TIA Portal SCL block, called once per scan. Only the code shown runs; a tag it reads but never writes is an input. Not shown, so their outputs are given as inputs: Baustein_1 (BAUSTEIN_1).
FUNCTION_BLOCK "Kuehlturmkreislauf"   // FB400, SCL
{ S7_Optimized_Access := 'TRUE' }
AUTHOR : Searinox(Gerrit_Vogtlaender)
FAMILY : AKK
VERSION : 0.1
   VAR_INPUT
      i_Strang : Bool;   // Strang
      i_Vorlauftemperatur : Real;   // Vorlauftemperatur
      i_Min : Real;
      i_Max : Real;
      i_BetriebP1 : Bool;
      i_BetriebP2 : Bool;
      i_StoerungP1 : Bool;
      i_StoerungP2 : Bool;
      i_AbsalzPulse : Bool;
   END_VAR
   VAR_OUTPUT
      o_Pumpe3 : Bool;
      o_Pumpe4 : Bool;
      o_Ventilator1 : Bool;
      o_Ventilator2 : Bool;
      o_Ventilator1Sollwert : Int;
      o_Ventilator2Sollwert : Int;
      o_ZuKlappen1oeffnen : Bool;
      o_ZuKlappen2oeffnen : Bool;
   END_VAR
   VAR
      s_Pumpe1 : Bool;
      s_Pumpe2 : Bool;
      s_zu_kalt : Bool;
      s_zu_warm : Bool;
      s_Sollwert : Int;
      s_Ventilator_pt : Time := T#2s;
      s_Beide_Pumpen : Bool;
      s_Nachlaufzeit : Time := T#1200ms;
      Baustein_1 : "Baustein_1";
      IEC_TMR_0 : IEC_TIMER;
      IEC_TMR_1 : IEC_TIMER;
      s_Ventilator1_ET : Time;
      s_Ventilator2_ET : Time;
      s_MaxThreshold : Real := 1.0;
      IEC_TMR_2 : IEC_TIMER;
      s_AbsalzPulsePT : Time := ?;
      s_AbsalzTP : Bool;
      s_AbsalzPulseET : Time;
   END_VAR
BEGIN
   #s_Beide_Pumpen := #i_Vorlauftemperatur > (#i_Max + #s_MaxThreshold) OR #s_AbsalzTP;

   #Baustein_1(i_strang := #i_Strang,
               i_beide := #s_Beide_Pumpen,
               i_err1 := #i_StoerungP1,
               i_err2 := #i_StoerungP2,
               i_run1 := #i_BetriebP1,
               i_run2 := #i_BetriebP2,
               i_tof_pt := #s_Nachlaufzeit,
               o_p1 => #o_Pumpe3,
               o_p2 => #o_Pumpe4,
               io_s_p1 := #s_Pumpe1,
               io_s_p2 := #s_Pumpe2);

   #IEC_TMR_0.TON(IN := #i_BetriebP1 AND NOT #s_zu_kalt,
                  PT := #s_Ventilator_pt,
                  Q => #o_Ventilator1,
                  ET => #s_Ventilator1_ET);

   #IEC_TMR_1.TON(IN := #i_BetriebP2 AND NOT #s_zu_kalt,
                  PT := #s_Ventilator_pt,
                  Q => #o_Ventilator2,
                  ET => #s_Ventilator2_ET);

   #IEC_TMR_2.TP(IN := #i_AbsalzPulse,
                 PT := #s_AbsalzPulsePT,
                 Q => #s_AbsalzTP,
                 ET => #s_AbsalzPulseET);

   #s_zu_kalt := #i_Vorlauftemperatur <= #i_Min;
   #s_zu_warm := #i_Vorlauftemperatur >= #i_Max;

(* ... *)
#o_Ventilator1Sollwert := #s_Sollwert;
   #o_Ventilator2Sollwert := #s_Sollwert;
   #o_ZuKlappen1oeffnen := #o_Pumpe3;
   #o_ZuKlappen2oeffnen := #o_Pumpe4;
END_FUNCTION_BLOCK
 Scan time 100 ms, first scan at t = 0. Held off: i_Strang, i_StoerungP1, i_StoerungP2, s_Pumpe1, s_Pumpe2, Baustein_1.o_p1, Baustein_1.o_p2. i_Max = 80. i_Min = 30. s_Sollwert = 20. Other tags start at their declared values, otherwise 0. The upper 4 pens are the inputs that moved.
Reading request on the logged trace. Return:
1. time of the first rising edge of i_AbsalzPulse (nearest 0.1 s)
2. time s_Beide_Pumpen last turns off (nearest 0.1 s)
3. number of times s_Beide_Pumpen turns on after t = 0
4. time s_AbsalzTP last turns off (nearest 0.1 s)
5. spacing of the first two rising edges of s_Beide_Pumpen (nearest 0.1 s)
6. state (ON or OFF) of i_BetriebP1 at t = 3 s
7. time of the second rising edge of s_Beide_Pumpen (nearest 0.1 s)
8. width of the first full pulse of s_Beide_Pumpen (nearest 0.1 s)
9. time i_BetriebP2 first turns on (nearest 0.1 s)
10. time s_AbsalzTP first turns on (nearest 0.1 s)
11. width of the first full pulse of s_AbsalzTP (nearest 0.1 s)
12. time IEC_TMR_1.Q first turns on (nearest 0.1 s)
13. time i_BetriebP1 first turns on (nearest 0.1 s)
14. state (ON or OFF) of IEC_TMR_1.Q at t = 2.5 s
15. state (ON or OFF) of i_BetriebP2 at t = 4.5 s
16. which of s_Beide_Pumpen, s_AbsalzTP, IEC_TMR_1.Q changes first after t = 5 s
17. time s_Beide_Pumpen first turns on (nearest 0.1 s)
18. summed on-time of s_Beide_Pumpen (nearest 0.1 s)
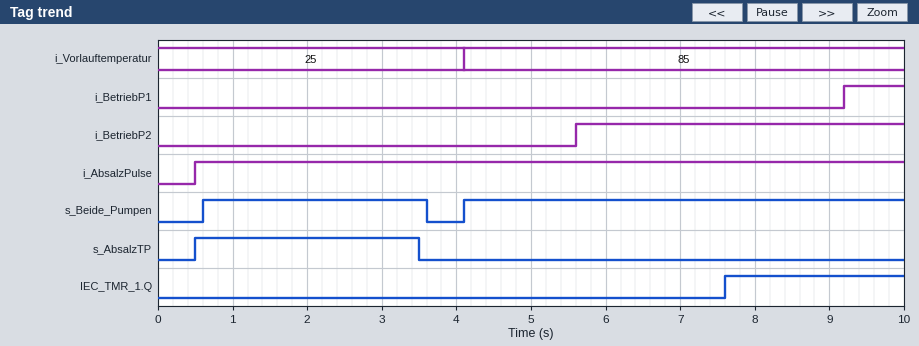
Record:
0.5 s
3.6 s
2
3.5 s
3.5 s
OFF
4.1 s
3.0 s
5.6 s
0.5 s
3.0 s
7.6 s
9.2 s
OFF
OFF
IEC_TMR_1.Q
0.6 s
8.9 s
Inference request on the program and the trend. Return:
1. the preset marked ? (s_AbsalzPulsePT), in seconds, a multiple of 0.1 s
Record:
3.0 s
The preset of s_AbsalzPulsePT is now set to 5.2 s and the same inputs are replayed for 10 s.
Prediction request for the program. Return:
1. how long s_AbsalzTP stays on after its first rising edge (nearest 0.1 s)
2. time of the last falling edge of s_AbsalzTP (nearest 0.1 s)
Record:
5.2 s
5.7 s
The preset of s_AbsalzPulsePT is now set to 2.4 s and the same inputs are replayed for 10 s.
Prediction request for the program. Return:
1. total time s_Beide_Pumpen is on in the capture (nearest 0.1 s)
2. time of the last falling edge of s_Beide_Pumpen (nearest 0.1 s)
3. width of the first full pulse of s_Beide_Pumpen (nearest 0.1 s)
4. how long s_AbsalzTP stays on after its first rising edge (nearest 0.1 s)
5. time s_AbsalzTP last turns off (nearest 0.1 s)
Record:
8.3 s
3.0 s
2.4 s
2.4 s
2.9 s
